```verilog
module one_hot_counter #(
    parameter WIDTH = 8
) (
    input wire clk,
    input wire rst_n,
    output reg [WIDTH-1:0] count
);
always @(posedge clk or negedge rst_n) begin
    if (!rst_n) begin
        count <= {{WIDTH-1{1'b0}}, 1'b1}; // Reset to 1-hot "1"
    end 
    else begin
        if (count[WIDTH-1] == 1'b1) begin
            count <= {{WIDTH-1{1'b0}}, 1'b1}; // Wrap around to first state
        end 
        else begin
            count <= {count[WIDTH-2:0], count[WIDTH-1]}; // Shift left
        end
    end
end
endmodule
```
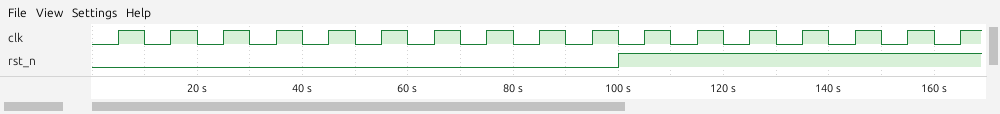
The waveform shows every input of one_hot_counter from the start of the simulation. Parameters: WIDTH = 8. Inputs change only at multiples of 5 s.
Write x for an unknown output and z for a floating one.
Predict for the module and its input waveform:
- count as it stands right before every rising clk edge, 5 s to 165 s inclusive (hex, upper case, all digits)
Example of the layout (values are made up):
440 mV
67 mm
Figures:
01, 01, 01, 01, 01, 01, 01, 01, 01, 01, 01, 02, 04, 08, 10, 20, 40
